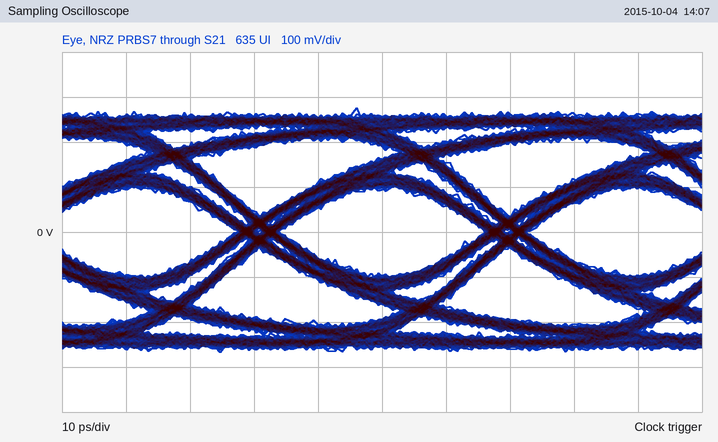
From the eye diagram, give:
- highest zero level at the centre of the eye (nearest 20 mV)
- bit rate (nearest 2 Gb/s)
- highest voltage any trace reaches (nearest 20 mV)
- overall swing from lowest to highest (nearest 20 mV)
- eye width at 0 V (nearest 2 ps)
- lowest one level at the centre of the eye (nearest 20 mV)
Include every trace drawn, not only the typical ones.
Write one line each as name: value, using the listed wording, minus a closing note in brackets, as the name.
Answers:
highest zero level at the centre of the eye: -100 mV
bit rate: 26 Gb/s
highest voltage any trace reaches: 280 mV
overall swing from lowest to highest: 540 mV
eye width at 0 V: 32 ps
lowest one level at the centre of the eye: 100 mV
